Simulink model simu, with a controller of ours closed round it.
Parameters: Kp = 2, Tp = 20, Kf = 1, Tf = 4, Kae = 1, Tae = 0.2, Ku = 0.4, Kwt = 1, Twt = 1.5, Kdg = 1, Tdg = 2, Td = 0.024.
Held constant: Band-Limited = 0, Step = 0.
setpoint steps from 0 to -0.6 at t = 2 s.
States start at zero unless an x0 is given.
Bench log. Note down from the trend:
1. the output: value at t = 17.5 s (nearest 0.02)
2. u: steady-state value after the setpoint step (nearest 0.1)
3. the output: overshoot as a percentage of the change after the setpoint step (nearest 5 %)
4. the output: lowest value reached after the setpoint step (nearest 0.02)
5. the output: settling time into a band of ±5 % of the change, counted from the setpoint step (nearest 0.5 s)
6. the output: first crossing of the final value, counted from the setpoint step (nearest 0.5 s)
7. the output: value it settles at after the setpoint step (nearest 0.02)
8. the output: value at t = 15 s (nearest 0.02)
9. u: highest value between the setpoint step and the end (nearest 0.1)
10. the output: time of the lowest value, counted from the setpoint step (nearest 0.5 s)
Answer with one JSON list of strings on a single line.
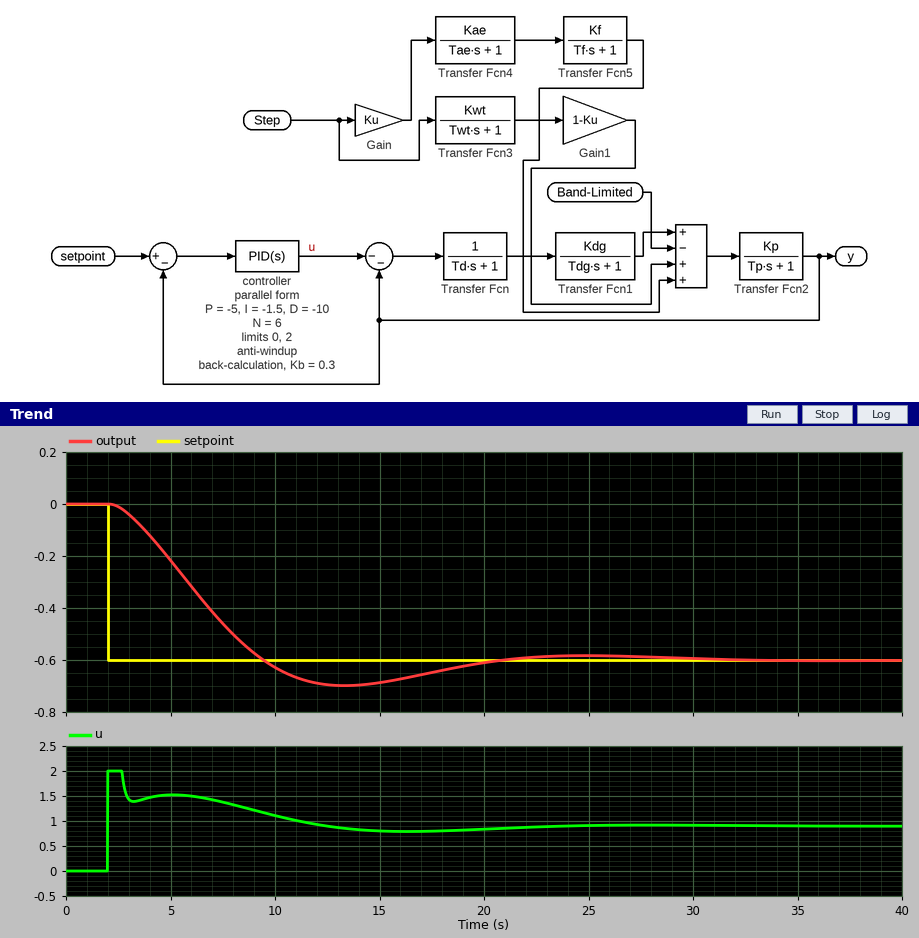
["-0.64", "0.9", "15 %", "-0.70", "16.5 s", "7.5 s", "-0.60", "-0.68", "2.0", "11.5 s"]
